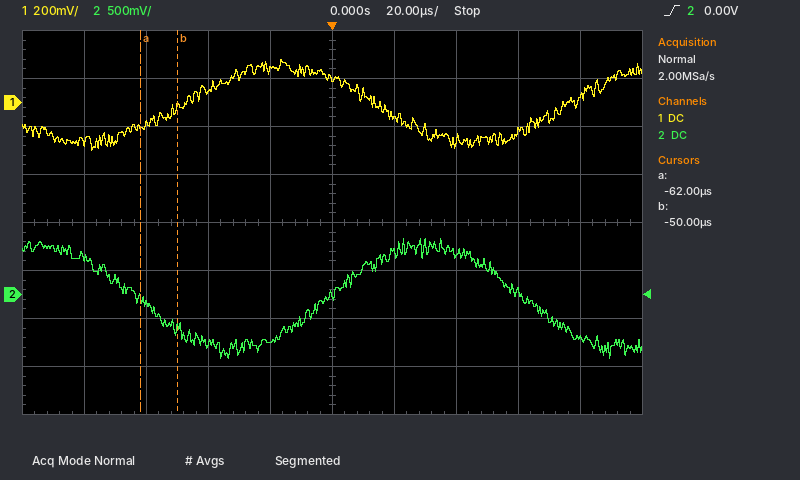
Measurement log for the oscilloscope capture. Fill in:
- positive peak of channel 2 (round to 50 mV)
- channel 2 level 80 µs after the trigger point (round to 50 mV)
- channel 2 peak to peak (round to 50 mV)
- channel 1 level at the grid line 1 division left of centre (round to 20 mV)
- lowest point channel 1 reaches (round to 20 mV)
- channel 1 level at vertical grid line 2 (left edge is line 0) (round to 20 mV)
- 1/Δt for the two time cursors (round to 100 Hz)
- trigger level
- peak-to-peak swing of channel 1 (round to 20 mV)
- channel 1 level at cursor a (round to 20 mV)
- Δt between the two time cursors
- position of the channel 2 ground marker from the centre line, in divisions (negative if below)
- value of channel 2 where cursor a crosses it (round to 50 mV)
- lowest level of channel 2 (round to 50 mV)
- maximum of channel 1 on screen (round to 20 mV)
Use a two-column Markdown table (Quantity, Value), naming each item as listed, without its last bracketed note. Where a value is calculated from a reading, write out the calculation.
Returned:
| Quantity | Value |
|---|---|
| positive peak of channel 2 | 600 mV |
| channel 2 level 80 µs after the trigger point | -450 mV |
| channel 2 peak to peak | 600 mV − (-650 mV) = 1.25 V |
| channel 1 level at the grid line 1 division left of centre | 140 mV |
| lowest point channel 1 reaches | -200 mV |
| channel 1 level at vertical grid line 2 (left edge is line 0) | -100 mV |
| 1/Δt for the two time cursors | 1 / 12 µs ≈ 83.3 kHz |
| trigger level | 0.00 V |
| peak-to-peak swing of channel 1 | 180 mV − (-200 mV) = 380 mV |
| channel 1 level at cursor a | -100 mV |
| Δt between the two time cursors | -50 µs − (-62 µs) = 12 µs |
| position of the channel 2 ground marker from the centre line, in divisions | -1.5 div |
| value of channel 2 where cursor a crosses it | -50 mV |
| lowest level of channel 2 | -650 mV |
| maximum of channel 1 on screen | 180 mV |
